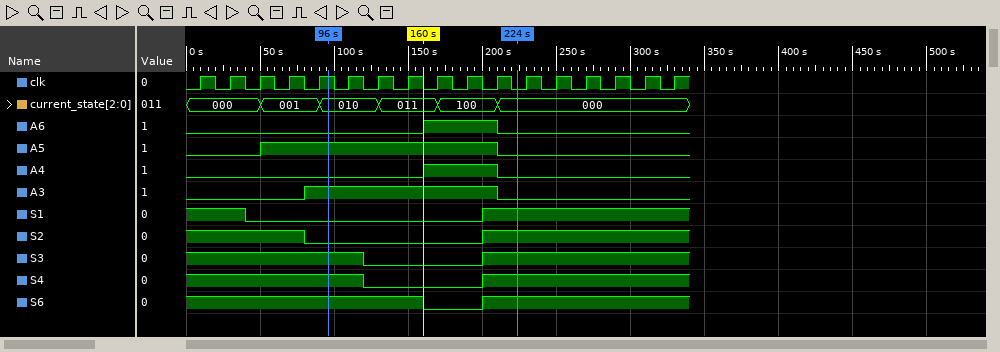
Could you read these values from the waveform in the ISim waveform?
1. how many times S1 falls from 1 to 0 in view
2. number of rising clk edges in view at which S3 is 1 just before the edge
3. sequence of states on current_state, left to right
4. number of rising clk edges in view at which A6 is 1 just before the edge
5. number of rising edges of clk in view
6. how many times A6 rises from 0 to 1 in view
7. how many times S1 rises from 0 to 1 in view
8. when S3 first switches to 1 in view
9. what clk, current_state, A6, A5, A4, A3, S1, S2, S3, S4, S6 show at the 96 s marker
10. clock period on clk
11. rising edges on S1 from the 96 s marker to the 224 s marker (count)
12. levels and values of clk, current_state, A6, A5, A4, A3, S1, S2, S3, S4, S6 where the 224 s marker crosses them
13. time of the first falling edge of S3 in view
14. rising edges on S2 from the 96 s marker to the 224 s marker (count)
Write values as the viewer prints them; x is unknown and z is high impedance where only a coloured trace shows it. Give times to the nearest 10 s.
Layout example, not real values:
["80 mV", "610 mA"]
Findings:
["1", "13", "000, 001, 010, 011, 100, 000", "3", "17", "1", "1", "200 s", "clk=1, current_state=010, A6=0, A5=1, A4=0, A3=1, S1=0, S2=0, S3=1, S4=1, S6=1", "20 s", "1", "clk=0, current_state=000, A6=0, A5=0, A4=0, A3=0, S1=1, S2=1, S3=1, S4=1, S6=1", "120 s", "1"]
